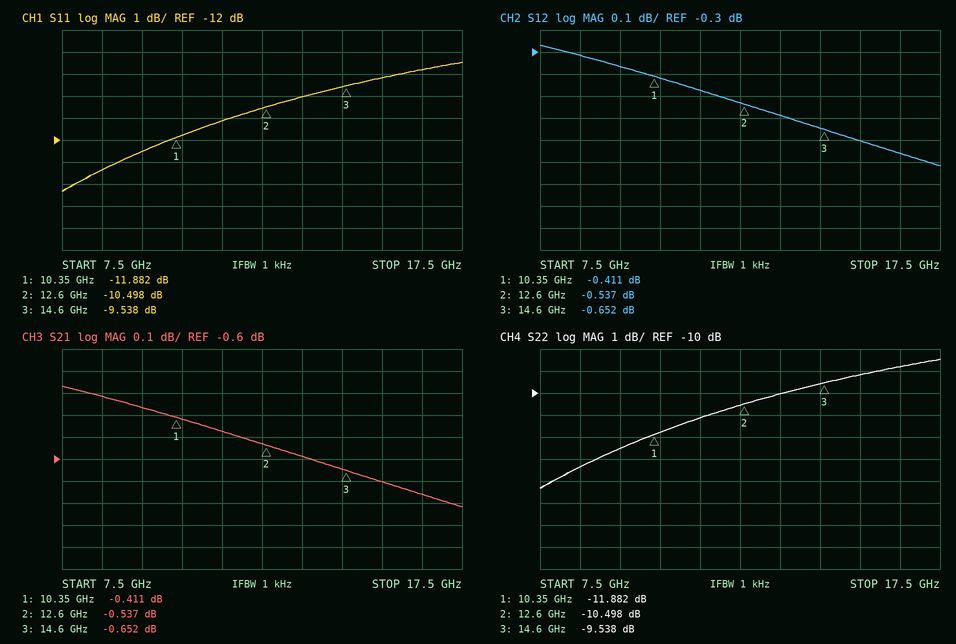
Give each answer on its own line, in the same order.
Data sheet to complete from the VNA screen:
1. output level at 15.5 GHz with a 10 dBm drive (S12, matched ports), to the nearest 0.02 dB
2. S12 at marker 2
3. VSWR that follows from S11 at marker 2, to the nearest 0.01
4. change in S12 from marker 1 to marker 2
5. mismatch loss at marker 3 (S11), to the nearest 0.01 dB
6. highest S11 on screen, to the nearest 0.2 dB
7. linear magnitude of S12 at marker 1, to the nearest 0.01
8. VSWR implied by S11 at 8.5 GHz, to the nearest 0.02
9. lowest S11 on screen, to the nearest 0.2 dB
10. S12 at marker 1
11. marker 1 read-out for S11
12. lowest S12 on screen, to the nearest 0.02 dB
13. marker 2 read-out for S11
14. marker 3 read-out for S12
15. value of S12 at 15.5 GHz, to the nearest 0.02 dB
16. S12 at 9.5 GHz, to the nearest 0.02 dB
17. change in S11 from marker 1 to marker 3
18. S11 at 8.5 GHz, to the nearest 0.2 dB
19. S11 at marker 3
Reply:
9.30 dBm
-0.537 dB
1.85
-0.126 dB
0.51 dB
-8.4 dB
0.95
1.54
-14.4 dB
-0.411 dB
-11.882 dB
-0.82 dB
-10.498 dB
-0.652 dB
-0.70 dB
-0.36 dB
2.344 dB
-13.4 dB
-9.538 dB
